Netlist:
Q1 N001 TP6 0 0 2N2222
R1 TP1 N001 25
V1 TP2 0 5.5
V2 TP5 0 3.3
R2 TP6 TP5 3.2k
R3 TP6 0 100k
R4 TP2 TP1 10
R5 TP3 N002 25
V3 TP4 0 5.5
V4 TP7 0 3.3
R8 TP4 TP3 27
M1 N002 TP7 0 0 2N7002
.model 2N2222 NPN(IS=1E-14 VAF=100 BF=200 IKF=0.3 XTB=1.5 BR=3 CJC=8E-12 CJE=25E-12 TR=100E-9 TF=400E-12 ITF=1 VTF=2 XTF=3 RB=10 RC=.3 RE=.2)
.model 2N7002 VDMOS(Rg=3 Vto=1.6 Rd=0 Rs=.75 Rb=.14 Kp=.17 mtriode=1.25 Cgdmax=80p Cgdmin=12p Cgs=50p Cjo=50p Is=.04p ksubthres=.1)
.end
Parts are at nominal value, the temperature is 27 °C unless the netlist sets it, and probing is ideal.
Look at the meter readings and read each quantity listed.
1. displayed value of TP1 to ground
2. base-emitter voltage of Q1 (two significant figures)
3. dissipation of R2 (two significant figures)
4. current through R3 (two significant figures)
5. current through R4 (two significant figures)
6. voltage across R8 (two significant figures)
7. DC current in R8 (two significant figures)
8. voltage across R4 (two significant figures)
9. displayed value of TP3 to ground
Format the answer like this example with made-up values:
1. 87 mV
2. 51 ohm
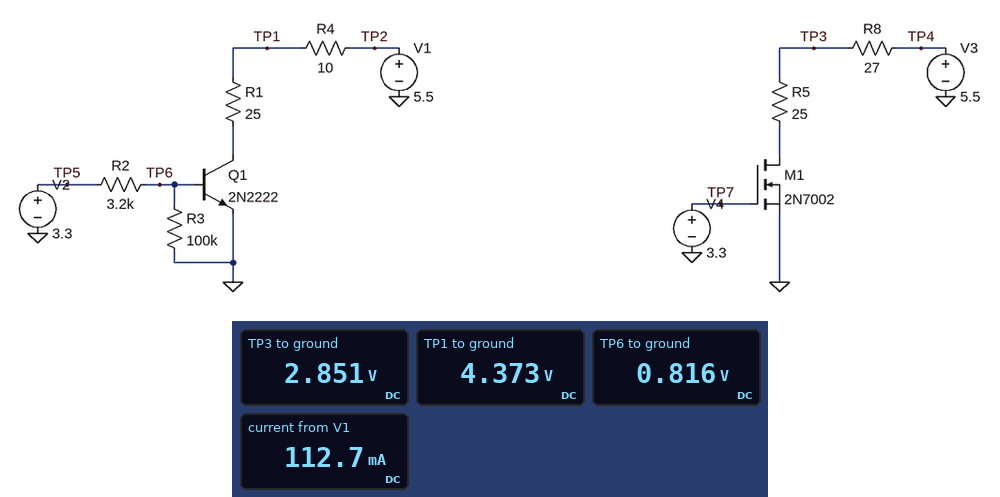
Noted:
1. 4.373 V
2. 820 mV
3. 1.9 mW
4. 8.2 µA
5. 110 mA
6. 2.6 V
7. 98 mA
8. 1.1 V
9. 2.851 V
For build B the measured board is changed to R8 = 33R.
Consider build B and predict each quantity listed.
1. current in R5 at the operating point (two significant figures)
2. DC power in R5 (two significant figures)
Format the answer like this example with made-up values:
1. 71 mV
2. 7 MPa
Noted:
1. 89 mA
2. 200 mW
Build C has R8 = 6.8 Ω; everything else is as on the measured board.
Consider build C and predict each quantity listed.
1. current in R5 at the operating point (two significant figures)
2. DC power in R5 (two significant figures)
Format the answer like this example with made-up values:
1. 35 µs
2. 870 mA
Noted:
1. 150 mA
2. 570 mW
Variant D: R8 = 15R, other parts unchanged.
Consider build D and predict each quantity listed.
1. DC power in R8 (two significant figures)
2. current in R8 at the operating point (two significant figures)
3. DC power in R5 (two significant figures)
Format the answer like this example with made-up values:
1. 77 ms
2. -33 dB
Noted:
1. 230 mW
2. 120 mA
3. 390 mW
